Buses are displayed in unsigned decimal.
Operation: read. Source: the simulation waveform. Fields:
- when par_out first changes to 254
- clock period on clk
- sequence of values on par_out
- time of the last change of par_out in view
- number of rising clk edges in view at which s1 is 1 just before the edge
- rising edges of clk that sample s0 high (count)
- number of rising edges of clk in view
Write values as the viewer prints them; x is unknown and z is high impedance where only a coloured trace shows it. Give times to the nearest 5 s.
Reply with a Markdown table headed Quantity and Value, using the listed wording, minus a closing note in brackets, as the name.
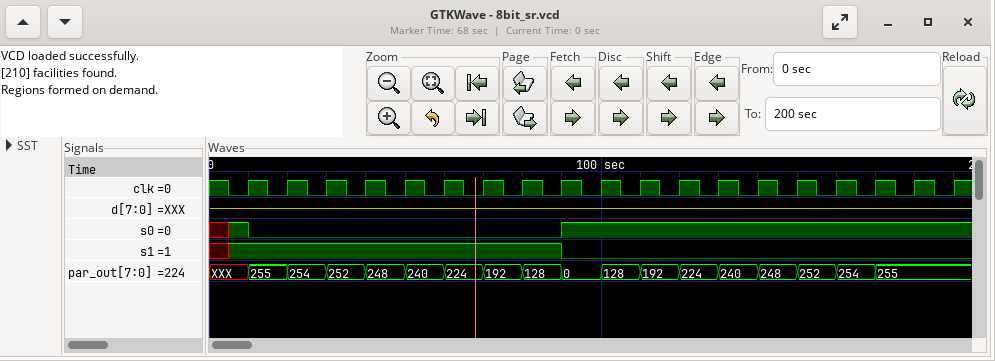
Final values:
| Quantity | Value |
|---|---|
| when par_out first changes to 254 | 20 s |
| clock period on clk | 10 s |
| sequence of values on par_out | XXX, 255, 254, 252, 248, 240, 224, 192, 128, 0, 128, 192, 224, 240, 248, 252, 254, 255 |
| time of the last change of par_out in view | 170 s |
| number of rising clk edges in view at which s1 is 1 just before the edge | 9 |
| rising edges of clk that sample s0 high | 11 |
| number of rising edges of clk in view | 19 |
